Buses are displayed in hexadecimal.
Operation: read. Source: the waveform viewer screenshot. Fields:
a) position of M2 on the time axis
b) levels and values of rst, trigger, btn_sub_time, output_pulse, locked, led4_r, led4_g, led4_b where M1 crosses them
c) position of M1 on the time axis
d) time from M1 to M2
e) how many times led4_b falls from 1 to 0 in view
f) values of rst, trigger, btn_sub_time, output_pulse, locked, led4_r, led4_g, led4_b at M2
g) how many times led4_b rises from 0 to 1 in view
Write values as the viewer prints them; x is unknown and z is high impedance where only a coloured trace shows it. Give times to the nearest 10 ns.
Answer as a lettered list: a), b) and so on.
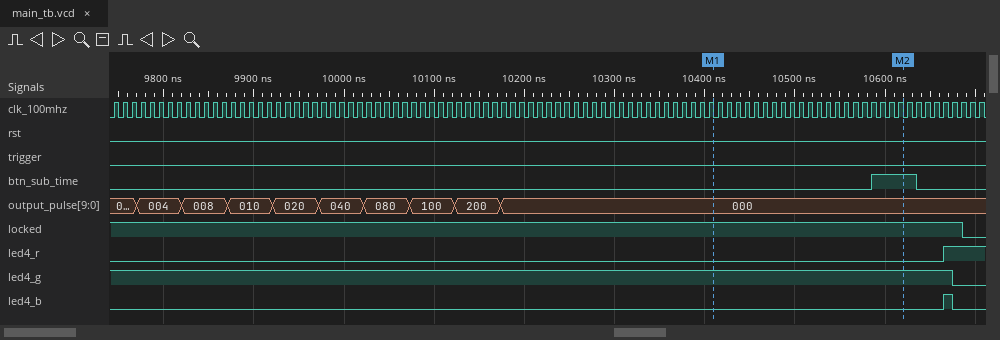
a) 10620 ns
b) rst=0, trigger=0, btn_sub_time=0, output_pulse=000, locked=1, led4_r=0, led4_g=1, led4_b=0
c) 10410 ns
d) 210 ns
e) 1
f) rst=0, trigger=0, btn_sub_time=1, output_pulse=000, locked=1, led4_r=0, led4_g=1, led4_b=0
g) 1
